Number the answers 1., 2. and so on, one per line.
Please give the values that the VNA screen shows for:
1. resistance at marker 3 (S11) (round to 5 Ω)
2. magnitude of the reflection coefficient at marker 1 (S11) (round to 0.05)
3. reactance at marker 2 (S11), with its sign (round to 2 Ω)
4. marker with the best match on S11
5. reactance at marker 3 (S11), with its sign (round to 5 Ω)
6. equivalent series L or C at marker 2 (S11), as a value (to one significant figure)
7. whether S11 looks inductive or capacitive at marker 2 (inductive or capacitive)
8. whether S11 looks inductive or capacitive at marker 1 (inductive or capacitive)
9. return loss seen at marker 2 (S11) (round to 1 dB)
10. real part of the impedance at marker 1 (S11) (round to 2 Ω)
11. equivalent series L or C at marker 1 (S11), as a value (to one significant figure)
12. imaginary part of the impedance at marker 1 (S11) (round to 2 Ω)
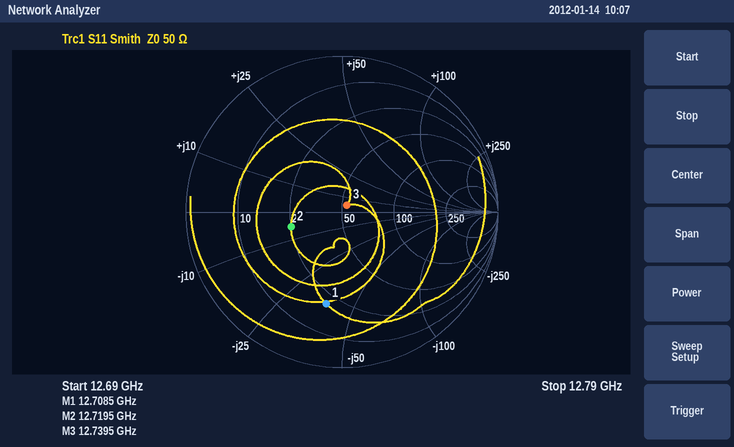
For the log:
1. 55 Ω
2. 0.60
3. -6 Ω
4. marker 3
5. +5 Ω
6. 2 pF
7. capacitive
8. capacitive
9. 9 dB
10. 20 Ω
11. 300 fF
12. -38 Ω
